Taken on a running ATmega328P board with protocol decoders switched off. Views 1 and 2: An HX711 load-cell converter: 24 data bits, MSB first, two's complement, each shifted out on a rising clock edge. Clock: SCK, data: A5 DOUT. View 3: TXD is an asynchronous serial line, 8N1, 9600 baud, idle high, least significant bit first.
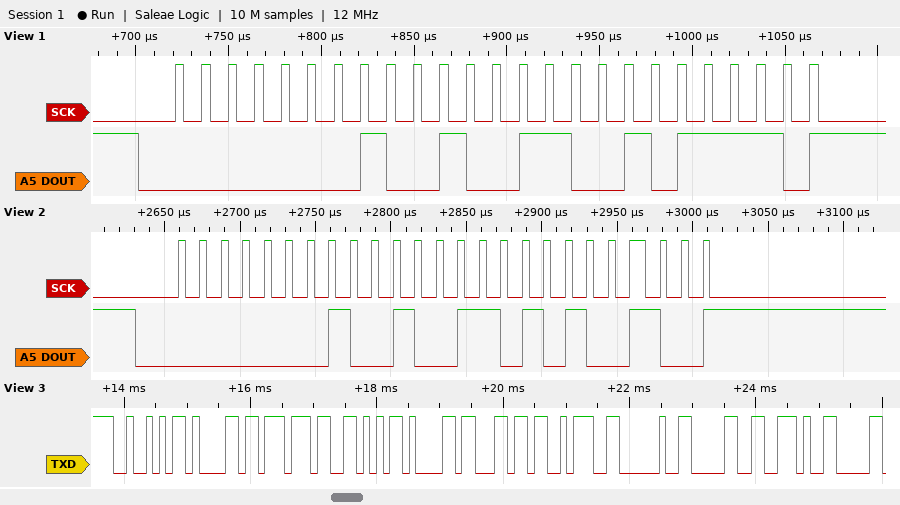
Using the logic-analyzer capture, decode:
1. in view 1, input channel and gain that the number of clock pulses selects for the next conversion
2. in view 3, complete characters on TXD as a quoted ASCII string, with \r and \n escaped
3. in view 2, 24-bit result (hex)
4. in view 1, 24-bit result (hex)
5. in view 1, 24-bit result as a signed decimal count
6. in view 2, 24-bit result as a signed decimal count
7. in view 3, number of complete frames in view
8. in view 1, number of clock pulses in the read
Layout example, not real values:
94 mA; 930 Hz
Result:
channel A, gain 128; "RawVal: 0."; 0x0126A4; 0x01265E; 75358; 75428; 10; 25
